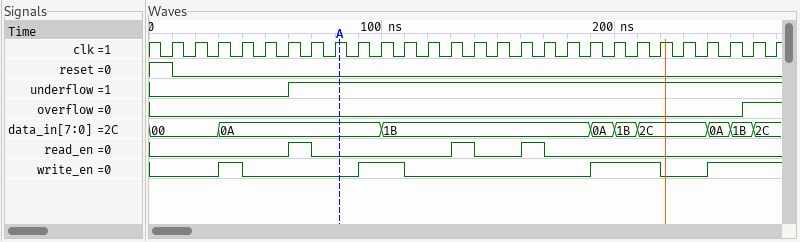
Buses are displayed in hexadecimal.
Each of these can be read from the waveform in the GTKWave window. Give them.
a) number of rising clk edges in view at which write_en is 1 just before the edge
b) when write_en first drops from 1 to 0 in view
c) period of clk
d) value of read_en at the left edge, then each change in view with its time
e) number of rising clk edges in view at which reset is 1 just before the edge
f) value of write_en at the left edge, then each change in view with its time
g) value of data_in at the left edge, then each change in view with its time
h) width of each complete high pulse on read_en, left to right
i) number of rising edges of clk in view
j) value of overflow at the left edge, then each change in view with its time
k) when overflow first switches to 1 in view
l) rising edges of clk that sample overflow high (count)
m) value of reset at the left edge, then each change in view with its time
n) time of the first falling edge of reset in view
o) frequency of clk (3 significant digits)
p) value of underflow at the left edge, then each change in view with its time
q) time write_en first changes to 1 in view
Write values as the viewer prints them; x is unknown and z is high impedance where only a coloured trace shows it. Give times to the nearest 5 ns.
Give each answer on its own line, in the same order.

9
40 ns
10 ns
0, 1 at 60 ns, 0 at 70 ns, 1 at 130 ns, 0 at 140 ns, 1 at 160 ns, 0 at 170 ns
1
0, 1 at 30 ns, 0 at 40 ns, 1 at 90 ns, 0 at 110 ns, 1 at 190 ns, 0 at 220 ns, 1 at 240 ns
00, 0A at 30 ns, 1B at 100 ns, 0A at 190 ns, 1B at 200 ns, 2C at 210 ns, 0A at 240 ns, 1B at 250 ns, 2C at 260 ns
10 ns, 10 ns, 10 ns
27
0, 1 at 255 ns
255 ns
2
1, 0 at 10 ns
10 ns
100 MHz
0, 1 at 60 ns
30 ns
